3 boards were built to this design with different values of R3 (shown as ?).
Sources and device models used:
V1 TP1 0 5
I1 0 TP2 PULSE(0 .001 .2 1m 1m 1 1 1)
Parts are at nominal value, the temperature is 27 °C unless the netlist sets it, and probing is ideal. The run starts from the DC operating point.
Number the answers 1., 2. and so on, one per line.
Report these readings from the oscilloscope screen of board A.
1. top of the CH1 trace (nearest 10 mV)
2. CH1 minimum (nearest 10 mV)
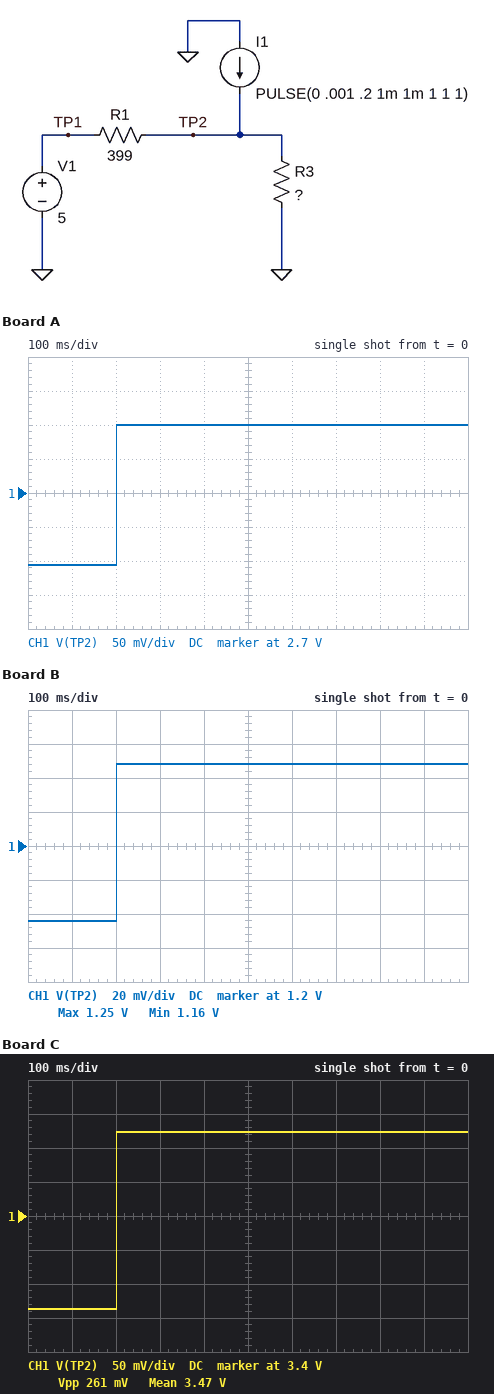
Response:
1. 2.80 V
2. 2.59 V
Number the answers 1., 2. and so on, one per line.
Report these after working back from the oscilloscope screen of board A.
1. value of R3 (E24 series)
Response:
1. 430 Ω
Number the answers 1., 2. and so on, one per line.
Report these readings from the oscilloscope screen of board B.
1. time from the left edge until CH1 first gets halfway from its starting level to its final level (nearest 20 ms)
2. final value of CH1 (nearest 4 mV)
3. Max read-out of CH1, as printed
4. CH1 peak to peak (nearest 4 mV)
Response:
1. 200 ms
2. 1.248 V
3. 1.25 V
4. 92 mV
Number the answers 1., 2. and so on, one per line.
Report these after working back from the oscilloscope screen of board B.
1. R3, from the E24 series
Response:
1. 120 Ω
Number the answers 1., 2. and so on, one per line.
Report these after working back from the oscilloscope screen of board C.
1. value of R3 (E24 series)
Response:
1. 750 Ω
